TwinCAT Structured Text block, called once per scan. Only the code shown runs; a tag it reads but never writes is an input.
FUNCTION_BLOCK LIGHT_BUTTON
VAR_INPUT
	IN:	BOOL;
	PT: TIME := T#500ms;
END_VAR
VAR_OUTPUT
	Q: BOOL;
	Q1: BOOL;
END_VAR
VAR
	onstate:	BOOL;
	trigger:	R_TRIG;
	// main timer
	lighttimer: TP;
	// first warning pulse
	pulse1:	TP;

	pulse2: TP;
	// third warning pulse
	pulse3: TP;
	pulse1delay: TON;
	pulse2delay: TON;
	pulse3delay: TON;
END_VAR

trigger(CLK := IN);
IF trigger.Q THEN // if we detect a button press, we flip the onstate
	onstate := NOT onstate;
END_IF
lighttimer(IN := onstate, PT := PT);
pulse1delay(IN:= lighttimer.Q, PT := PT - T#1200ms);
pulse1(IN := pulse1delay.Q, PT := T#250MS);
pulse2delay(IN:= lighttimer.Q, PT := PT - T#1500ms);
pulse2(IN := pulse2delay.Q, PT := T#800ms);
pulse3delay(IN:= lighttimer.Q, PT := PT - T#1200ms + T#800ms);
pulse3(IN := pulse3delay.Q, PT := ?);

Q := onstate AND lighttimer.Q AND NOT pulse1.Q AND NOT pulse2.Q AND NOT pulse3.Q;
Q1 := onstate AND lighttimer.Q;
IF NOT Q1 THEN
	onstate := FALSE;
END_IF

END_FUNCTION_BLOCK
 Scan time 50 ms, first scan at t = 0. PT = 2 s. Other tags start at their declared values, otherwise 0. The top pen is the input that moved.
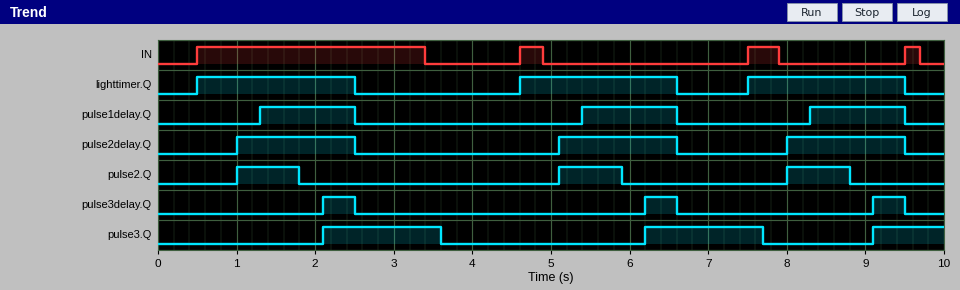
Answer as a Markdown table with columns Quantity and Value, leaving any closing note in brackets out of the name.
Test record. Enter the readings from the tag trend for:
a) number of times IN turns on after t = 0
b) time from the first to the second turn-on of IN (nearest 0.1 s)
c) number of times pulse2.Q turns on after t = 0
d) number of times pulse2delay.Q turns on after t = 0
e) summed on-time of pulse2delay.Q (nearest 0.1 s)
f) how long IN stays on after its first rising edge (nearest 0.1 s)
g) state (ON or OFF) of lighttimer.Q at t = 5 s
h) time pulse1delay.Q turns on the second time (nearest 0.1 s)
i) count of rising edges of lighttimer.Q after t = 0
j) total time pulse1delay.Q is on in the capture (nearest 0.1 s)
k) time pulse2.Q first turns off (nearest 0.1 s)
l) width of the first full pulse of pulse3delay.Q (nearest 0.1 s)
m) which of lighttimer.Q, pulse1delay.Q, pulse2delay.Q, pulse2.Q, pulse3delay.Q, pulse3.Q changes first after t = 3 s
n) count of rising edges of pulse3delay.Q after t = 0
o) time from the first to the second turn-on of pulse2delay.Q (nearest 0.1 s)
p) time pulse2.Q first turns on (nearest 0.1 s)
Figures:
| Quantity | Value |
|---|---|
| number of times IN turns on after t = 0 | 4 |
| time from the first to the second turn-on of IN | 4.1 s |
| number of times pulse2.Q turns on after t = 0 | 3 |
| number of times pulse2delay.Q turns on after t = 0 | 3 |
| summed on-time of pulse2delay.Q | 4.5 s |
| how long IN stays on after its first rising edge | 2.9 s |
| state (ON or OFF) of lighttimer.Q at t = 5 s | ON |
| time pulse1delay.Q turns on the second time | 5.4 s |
| count of rising edges of lighttimer.Q after t = 0 | 3 |
| total time pulse1delay.Q is on in the capture | 3.6 s |
| time pulse2.Q first turns off | 1.8 s |
| width of the first full pulse of pulse3delay.Q | 0.4 s |
| which of lighttimer.Q, pulse1delay.Q, pulse2delay.Q, pulse2.Q, pulse3delay.Q, pulse3.Q changes first after t = 3 s | pulse3.Q |
| count of rising edges of pulse3delay.Q after t = 0 | 3 |
| time from the first to the second turn-on of pulse2delay.Q | 4.1 s |
| time pulse2.Q first turns on | 1.0 s |
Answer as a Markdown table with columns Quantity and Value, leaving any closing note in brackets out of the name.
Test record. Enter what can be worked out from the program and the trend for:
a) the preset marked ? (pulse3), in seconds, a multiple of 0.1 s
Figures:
| Quantity | Value |
|---|---|
| the preset marked ? (pulse3), in seconds, a multiple of 0.1 s | 1.5 s |
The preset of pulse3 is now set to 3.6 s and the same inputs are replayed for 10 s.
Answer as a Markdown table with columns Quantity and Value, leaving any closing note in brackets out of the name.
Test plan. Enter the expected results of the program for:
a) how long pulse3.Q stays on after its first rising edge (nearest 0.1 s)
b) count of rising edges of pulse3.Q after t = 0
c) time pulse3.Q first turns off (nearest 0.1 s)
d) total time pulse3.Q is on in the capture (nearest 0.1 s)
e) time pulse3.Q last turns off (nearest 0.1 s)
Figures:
| Quantity | Value |
|---|---|
| how long pulse3.Q stays on after its first rising edge | 3.6 s |
| count of rising edges of pulse3.Q after t = 0 | 2 |
| time pulse3.Q first turns off | 5.7 s |
| total time pulse3.Q is on in the capture | 7.2 s |
| time pulse3.Q last turns off | 9.8 s |
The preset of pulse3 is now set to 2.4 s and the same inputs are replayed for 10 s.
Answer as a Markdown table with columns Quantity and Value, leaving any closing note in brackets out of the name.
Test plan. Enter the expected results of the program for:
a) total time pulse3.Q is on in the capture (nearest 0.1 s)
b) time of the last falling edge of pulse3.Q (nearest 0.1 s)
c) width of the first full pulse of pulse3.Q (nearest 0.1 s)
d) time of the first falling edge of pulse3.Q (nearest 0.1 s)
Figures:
| Quantity | Value |
|---|---|
| total time pulse3.Q is on in the capture | 5.7 s |
| time of the last falling edge of pulse3.Q | 8.6 s |
| width of the first full pulse of pulse3.Q | 2.4 s |
| time of the first falling edge of pulse3.Q | 4.5 s |
